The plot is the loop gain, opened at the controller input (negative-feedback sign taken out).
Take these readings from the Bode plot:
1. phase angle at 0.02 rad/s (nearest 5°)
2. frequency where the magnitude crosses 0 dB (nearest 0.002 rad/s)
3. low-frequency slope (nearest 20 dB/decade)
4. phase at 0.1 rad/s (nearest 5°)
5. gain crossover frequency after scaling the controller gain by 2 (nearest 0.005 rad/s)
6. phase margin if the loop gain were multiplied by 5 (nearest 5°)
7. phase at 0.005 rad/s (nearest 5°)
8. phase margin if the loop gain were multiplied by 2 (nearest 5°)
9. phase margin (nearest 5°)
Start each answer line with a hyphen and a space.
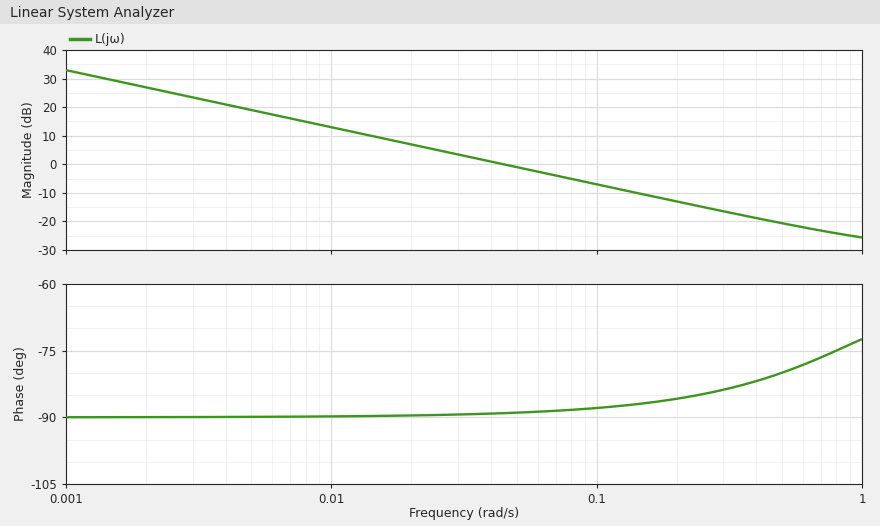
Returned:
- -90°
- 0.044 rad/s
- -20 dB/decade
- -90°
- 0.090 rad/s
- 95°
- -90°
- 90°
- 90°
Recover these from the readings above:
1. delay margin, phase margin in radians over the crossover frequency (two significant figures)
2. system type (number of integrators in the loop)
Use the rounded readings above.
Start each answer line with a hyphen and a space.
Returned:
- 36 s
- 1
